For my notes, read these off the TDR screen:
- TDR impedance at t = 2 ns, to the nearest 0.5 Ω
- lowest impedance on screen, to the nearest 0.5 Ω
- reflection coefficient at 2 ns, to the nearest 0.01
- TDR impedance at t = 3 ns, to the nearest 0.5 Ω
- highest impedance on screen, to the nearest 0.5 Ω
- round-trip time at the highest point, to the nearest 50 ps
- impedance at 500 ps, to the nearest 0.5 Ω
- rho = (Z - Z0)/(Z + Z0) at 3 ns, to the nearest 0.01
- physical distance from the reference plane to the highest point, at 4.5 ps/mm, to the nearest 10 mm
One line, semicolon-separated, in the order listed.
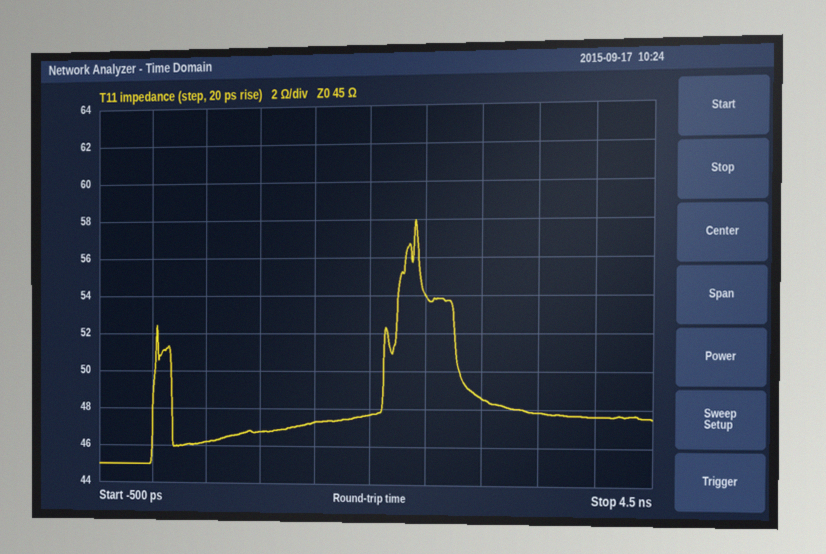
47.5 Ω; 45.0 Ω; +0.03; 48.5 Ω; 58.0 Ω; 2.40 ns; 46.0 Ω; +0.04; 270 mm
